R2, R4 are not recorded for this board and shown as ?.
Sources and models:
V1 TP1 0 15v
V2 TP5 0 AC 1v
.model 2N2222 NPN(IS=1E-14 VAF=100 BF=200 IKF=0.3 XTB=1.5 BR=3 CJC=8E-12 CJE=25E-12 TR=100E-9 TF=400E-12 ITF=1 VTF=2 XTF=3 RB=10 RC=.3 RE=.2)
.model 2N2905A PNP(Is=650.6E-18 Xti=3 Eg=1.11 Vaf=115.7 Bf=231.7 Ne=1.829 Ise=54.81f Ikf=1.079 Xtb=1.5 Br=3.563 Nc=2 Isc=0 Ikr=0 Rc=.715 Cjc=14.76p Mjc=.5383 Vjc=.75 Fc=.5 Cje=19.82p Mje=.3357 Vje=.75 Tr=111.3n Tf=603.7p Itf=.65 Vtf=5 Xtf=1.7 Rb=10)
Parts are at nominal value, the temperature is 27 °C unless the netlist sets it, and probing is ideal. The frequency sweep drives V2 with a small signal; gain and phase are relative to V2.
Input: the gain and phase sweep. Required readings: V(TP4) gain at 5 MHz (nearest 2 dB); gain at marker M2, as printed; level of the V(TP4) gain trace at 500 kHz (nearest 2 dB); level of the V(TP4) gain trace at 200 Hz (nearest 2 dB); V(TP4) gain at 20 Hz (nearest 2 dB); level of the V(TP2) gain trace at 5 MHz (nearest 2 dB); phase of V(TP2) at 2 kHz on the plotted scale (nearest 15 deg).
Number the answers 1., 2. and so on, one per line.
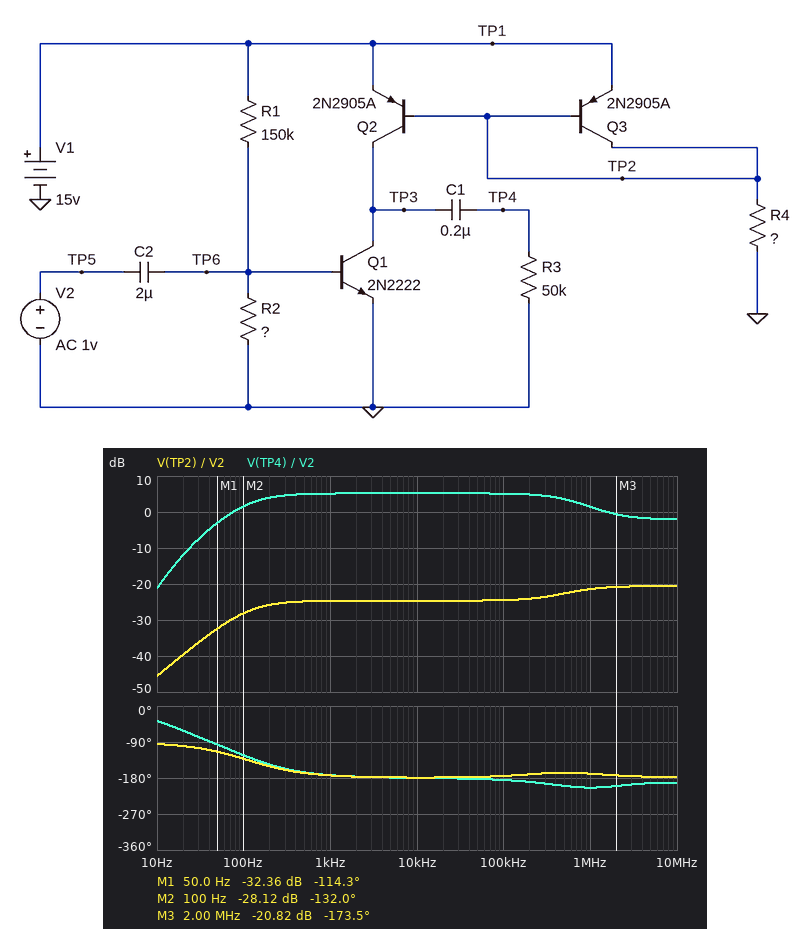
1. -2 dB
2. -28.12 dB
3. 4 dB
4. 4 dB
5. -12 dB
6. -20 dB
7. -180 deg
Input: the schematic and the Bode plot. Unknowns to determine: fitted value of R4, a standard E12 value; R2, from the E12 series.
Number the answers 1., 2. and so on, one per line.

1. 1 kΩ
2. 12 kΩ
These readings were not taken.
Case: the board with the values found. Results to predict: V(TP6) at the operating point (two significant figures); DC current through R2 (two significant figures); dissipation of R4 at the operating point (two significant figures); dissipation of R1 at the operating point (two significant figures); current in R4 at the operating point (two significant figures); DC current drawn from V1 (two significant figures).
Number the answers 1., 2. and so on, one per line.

1. 710 mV
2. 59 µA
3. 200 mW
4. 1.4 mW
5. 14 mA
6. 22 mA
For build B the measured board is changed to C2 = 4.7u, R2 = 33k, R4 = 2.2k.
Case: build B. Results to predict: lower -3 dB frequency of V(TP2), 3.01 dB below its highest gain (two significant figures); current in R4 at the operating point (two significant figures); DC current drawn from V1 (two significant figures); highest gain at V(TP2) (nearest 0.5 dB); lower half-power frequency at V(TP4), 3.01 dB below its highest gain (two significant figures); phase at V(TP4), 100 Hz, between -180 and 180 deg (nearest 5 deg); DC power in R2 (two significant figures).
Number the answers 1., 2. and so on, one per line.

1. 910 kHz
2. 6.5 mA
3. 14 mA
4. -54.5 dB
5. 1.4 kHz
6. -85 deg
7. 15 µW
